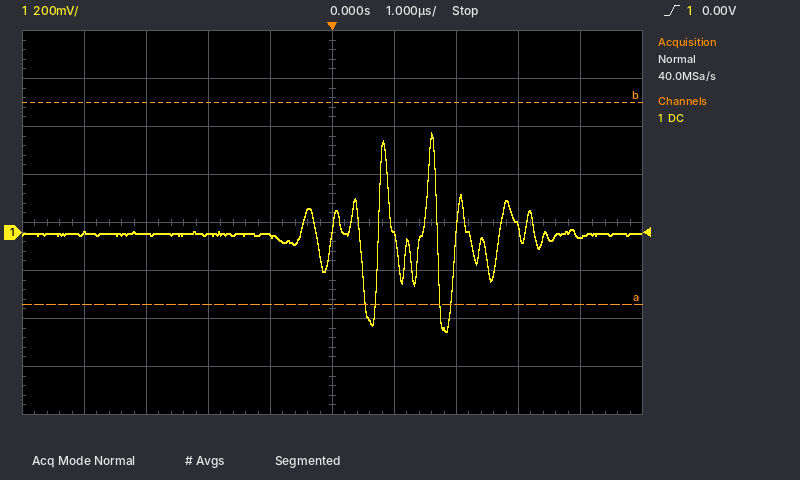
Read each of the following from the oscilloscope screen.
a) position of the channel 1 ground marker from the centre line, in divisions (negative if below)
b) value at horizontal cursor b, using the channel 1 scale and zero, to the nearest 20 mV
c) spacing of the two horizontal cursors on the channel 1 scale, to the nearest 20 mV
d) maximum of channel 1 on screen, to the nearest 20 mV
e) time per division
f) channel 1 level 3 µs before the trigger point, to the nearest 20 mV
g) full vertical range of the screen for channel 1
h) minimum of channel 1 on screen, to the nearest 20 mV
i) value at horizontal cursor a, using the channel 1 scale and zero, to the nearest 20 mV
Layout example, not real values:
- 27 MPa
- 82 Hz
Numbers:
- -0.2 div
- 540 mV
- 840 mV
- 420 mV
- 1 µs
- 0 mV
- 1.6 V
- -420 mV
- -300 mV
